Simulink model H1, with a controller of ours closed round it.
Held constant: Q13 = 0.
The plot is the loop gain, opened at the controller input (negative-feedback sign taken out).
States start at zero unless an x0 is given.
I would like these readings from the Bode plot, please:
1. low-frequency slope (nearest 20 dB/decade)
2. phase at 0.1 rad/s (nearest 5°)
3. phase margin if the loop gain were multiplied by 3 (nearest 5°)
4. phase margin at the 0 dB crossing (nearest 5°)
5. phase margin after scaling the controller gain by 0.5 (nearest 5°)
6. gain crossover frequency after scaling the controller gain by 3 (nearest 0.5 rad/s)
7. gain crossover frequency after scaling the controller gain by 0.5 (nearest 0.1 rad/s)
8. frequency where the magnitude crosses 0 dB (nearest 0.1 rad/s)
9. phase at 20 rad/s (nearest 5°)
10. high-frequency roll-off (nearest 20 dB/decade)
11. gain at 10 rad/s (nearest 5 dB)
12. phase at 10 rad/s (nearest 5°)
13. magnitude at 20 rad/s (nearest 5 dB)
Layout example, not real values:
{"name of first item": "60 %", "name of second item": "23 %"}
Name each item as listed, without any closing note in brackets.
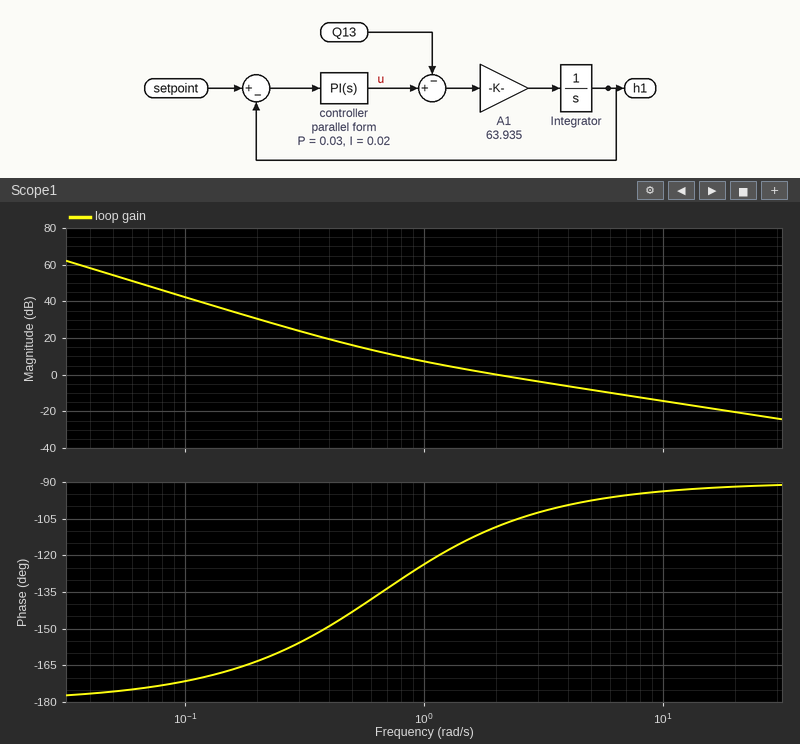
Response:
{"low-frequency slope": "-40 dB/decade", "phase at 0.1 rad/s": "-170°", "phase margin if the loop gain were multiplied by 3": "85°", "phase margin at the 0 dB crossing": "70°", "phase margin after scaling the controller gain by 0.5": "60°", "gain crossover frequency after scaling the controller gain by 3": "6.0 rad/s", "gain crossover frequency after scaling the controller gain by 0.5": "1.1 rad/s", "frequency where the magnitude crosses 0 dB": "2.0 rad/s", "phase at 20 rad/s": "-90°", "high-frequency roll-off": "-20 dB/decade", "gain at 10 rad/s": "-15 dB", "phase at 10 rad/s": "-95°", "magnitude at 20 rad/s": "-20 dB"}
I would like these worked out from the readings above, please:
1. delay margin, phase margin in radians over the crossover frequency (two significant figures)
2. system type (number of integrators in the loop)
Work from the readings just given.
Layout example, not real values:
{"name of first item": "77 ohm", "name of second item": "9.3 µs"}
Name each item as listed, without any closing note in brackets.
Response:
{"delay margin, phase margin in radians over the crossover frequency": "0.61 s", "system type": "2"}
